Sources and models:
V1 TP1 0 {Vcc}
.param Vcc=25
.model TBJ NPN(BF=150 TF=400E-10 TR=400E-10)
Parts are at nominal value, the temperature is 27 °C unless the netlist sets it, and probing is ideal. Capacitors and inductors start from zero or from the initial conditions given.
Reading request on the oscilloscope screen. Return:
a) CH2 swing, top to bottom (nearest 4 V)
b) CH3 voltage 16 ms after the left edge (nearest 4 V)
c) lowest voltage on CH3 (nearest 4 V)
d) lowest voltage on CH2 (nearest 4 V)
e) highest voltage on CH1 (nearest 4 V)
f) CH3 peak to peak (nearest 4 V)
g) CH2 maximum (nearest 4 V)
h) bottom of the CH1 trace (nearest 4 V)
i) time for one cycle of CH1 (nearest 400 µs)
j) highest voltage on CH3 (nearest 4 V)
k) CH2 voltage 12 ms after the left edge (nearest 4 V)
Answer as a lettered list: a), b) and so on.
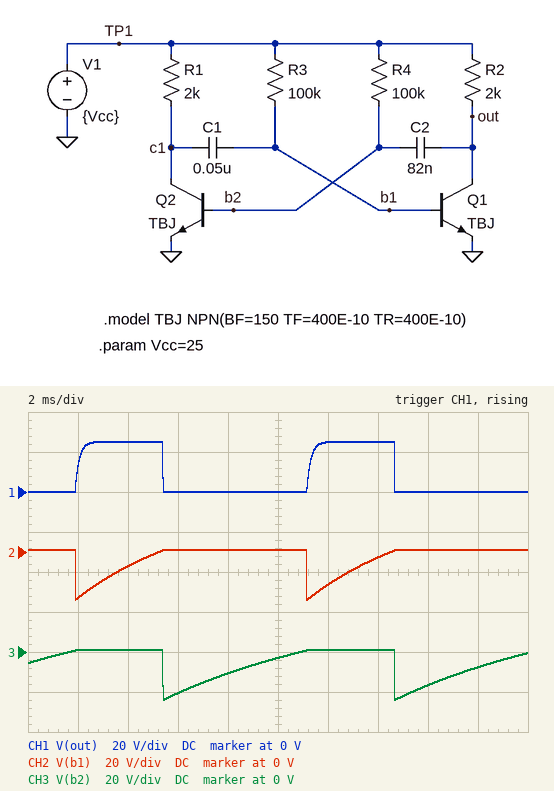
a) 24 V
b) -16 V
c) -24 V
d) -24 V
e) 24 V
f) 24 V
g) 0 V
h) 0 V
i) 9.2 ms
j) 0 V
k) -16 V
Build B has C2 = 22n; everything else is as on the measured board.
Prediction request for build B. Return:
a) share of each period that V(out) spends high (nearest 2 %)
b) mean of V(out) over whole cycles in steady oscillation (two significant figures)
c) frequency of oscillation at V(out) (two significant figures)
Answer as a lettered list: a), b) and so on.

a) 68 %
b) 17 V
c) 200 Hz
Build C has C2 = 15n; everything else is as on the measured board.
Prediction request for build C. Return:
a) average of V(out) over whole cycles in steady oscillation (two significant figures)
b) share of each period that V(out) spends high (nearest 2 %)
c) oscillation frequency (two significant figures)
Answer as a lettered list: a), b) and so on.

a) 19 V
b) 76 %
c) 220 Hz
